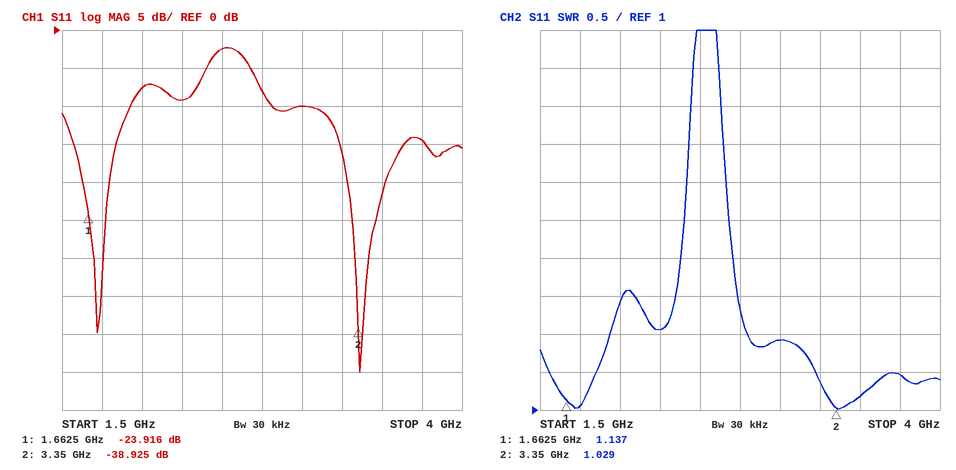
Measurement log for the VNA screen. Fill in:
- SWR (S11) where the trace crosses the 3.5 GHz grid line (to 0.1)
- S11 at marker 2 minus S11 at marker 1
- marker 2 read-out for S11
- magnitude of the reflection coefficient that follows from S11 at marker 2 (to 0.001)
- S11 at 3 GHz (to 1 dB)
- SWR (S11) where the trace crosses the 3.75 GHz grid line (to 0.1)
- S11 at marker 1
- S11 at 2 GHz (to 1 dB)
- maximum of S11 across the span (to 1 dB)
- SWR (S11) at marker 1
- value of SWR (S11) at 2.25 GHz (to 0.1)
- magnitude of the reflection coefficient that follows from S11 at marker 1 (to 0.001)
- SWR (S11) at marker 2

1.2
-15.009 dB
-38.925 dB
0.011
-10 dB
1.5
-23.916 dB
-8 dB
-2 dB
1.137
2.1
0.064
1.029
